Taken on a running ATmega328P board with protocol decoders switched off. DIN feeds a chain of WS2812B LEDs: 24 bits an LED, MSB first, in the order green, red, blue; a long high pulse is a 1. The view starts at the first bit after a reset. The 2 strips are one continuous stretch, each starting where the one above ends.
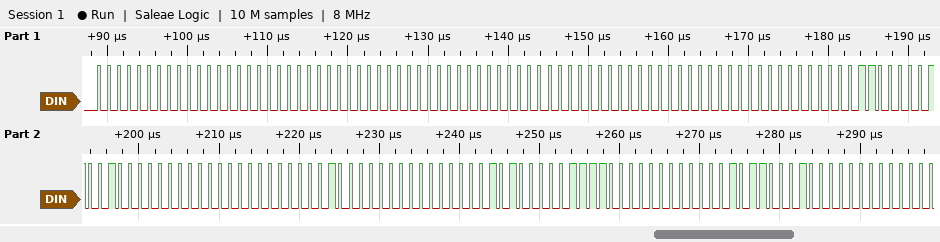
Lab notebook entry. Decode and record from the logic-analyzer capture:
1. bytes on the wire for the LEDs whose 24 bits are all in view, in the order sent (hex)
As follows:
00 00 00 00 00 00 00 00 00 0C 12 00 00 08 00 0A 0F 00 0B 10 00
